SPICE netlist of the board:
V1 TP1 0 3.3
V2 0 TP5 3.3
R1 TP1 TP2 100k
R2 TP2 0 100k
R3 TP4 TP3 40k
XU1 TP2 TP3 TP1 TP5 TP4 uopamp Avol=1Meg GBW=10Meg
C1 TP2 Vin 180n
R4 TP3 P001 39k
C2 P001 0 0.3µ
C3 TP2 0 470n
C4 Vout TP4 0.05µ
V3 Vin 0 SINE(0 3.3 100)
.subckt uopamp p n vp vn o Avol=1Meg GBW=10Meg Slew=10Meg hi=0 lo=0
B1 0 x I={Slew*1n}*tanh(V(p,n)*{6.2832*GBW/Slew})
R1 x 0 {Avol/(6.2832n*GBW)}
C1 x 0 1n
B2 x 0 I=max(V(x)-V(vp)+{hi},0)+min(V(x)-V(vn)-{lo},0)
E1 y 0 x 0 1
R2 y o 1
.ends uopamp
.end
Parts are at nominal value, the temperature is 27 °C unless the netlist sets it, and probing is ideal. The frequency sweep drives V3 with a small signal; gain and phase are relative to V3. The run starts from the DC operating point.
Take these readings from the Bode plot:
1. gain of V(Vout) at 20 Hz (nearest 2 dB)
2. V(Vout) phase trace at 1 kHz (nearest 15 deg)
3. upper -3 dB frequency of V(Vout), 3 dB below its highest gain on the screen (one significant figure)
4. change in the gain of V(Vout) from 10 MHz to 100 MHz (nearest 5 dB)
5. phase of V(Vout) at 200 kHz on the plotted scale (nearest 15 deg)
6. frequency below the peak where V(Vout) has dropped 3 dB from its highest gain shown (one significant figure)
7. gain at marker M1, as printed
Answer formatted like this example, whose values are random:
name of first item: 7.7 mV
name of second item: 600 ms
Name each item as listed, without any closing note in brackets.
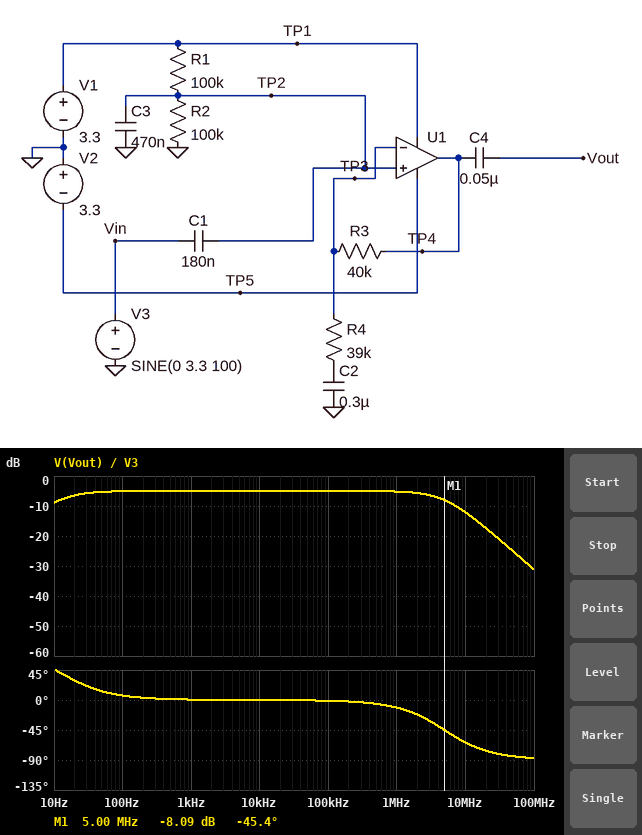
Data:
gain of V(Vout) at 20 Hz: -6 dB
V(Vout) phase trace at 1 kHz: 0 deg
upper -3 dB frequency of V(Vout), 3 dB below its highest gain on the screen: 5 MHz
change in the gain of V(Vout) from 10 MHz to 100 MHz: -20 dB
phase of V(Vout) at 200 kHz on the plotted scale: 0 deg
frequency below the peak where V(Vout) has dropped 3 dB from its highest gain shown: 10 Hz
gain at marker M1, as printed: -8.09 dB
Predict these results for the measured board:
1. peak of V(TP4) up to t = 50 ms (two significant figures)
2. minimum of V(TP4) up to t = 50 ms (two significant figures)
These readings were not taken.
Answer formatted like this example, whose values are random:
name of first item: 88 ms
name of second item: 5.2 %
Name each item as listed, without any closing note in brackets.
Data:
peak of V(TP4) up to t = 50 ms: 3.3 V
minimum of V(TP4) up to t = 50 ms: -310 mV
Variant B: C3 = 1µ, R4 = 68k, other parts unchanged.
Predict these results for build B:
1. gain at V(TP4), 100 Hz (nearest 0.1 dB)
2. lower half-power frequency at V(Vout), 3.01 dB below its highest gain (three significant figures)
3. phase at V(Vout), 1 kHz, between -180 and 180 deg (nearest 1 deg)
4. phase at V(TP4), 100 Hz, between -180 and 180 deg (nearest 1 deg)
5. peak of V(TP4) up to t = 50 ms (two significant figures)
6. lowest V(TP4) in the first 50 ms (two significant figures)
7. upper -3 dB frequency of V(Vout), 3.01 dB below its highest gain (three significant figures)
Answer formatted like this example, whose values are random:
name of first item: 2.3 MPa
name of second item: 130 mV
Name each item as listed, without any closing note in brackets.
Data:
gain at V(TP4), 100 Hz: -12.3 dB
lower half-power frequency at V(Vout), 3.01 dB below its highest gain: 5.76 Hz
phase at V(Vout), 1 kHz, between -180 and 180 deg: 0 deg
phase at V(TP4), 100 Hz, between -180 and 180 deg: 3 deg
peak of V(TP4) up to t = 50 ms: 2.4 V
lowest V(TP4) in the first 50 ms: 820 mV
upper -3 dB frequency of V(Vout), 3.01 dB below its highest gain: 6.30 MHz
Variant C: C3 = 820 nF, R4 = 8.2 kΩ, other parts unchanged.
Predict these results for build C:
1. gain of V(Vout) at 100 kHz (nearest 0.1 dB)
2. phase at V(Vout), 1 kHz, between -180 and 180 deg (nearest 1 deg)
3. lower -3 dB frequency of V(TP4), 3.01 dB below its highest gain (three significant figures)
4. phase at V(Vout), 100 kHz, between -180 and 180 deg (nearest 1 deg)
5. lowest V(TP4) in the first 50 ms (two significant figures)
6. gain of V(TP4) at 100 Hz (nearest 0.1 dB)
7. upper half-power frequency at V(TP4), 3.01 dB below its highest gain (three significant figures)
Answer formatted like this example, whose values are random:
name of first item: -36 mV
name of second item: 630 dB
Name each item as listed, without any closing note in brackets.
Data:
gain of V(Vout) at 100 kHz: 0.5 dB
phase at V(Vout), 1 kHz, between -180 and 180 deg: 3 deg
lower -3 dB frequency of V(TP4), 3.01 dB below its highest gain: 63.0 Hz
phase at V(Vout), 100 kHz, between -180 and 180 deg: -3 deg
lowest V(TP4) in the first 50 ms: -1.3 V
gain of V(TP4) at 100 Hz: -1.0 dB
upper half-power frequency at V(TP4), 3.01 dB below its highest gain: 1.70 MHz
